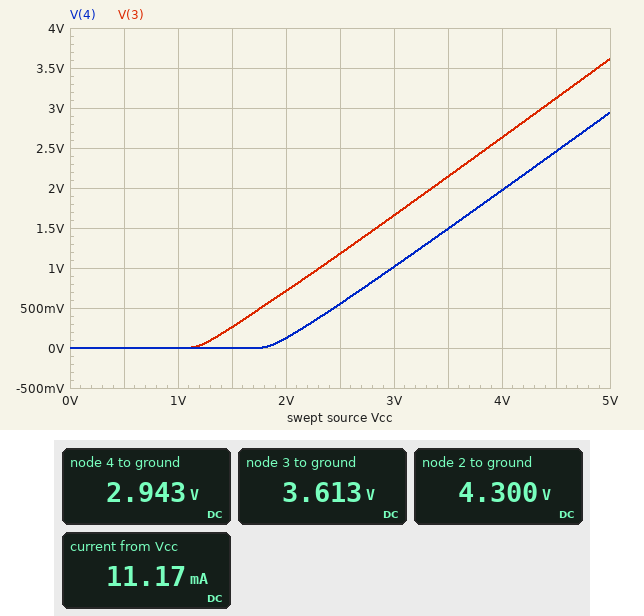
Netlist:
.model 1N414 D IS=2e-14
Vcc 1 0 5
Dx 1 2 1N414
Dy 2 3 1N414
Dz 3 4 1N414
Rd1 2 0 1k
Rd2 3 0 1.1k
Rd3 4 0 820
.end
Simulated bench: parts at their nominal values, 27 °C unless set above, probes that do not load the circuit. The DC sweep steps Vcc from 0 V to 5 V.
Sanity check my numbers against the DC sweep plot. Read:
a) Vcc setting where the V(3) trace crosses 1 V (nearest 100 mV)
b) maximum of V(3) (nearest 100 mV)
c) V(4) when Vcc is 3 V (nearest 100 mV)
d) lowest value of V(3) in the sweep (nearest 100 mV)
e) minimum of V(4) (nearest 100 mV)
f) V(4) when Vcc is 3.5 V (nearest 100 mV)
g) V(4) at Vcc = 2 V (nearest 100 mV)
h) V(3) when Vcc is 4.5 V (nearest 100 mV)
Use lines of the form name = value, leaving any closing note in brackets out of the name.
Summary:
Vcc setting where the V(3) trace crosses 1 V = 2.3 V
maximum of V(3) = 3.6 V
V(4) when Vcc is 3 V = 1.0 V
lowest value of V(3) in the sweep = 0 V
minimum of V(4) = 0 V
V(4) when Vcc is 3.5 V = 1.5 V
V(4) at Vcc = 2 V = 100 mV
V(3) when Vcc is 4.5 V = 3.1 V
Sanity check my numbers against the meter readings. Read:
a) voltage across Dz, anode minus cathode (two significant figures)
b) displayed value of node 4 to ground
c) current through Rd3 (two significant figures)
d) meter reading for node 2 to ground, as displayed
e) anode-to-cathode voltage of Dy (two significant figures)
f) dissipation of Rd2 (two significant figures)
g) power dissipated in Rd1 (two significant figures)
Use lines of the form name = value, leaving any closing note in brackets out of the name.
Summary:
voltage across Dz, anode minus cathode = 670 mV
displayed value of node 4 to ground = 2.943 V
current through Rd3 = 3.6 mA
meter reading for node 2 to ground, as displayed = 4.300 V
anode-to-cathode voltage of Dy = 690 mV
dissipation of Rd2 = 12 mW
power dissipated in Rd1 = 18 mW
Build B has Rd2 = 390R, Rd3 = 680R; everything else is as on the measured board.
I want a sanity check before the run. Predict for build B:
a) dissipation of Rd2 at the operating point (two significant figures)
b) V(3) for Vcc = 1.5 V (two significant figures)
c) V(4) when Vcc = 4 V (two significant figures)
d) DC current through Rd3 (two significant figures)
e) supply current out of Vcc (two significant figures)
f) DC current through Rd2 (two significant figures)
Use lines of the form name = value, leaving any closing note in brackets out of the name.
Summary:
dissipation of Rd2 at the operating point = 33 mW
V(3) for Vcc = 1.5 V = 230 mV
V(4) when Vcc = 4 V = 1.9 V
DC current through Rd3 = 4.3 mA
supply current out of Vcc = 18 mA
DC current through Rd2 = 9.2 mA
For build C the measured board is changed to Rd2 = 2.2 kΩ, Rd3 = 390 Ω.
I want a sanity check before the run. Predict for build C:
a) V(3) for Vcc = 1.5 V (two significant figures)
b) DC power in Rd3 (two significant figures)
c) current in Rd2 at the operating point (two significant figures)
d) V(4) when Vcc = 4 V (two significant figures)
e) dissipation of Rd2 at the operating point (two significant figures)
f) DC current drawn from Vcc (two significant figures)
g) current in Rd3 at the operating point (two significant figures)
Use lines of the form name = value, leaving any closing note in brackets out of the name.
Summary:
V(3) for Vcc = 1.5 V = 280 mV
DC power in Rd3 = 22 mW
current in Rd2 at the operating point = 1.6 mA
V(4) when Vcc = 4 V = 1.9 V
dissipation of Rd2 at the operating point = 5.9 mW
DC current drawn from Vcc = 13 mA
current in Rd3 at the operating point = 7.5 mA
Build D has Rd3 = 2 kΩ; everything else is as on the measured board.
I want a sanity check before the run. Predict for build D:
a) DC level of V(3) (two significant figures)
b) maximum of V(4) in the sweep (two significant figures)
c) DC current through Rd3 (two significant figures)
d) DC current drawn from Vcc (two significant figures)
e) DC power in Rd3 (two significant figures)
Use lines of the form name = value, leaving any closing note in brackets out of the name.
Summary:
DC level of V(3) = 3.6 V
maximum of V(4) in the sweep = 3.0 V
DC current through Rd3 = 1.5 mA
DC current drawn from Vcc = 9.1 mA
DC power in Rd3 = 4.4 mW
